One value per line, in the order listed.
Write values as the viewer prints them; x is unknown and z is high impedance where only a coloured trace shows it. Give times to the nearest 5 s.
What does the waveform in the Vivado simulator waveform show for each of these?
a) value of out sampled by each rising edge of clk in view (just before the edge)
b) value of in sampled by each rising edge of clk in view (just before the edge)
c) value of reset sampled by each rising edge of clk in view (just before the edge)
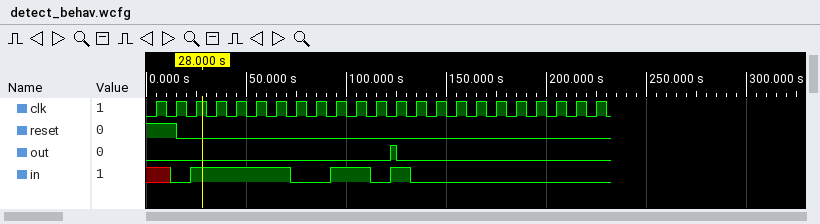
0 0 0 0 0 0 0 0 0 0 0 0 1 0 0 0 0 0 0 0 0 0 0
x 0 1 1 1 1 1 0 0 1 1 0 1 0 0 0 0 0 0 0 0 0 0
1 1 0 0 0 0 0 0 0 0 0 0 0 0 0 0 0 0 0 0 0 0 0
